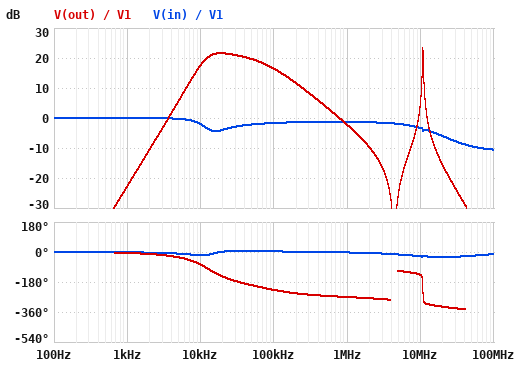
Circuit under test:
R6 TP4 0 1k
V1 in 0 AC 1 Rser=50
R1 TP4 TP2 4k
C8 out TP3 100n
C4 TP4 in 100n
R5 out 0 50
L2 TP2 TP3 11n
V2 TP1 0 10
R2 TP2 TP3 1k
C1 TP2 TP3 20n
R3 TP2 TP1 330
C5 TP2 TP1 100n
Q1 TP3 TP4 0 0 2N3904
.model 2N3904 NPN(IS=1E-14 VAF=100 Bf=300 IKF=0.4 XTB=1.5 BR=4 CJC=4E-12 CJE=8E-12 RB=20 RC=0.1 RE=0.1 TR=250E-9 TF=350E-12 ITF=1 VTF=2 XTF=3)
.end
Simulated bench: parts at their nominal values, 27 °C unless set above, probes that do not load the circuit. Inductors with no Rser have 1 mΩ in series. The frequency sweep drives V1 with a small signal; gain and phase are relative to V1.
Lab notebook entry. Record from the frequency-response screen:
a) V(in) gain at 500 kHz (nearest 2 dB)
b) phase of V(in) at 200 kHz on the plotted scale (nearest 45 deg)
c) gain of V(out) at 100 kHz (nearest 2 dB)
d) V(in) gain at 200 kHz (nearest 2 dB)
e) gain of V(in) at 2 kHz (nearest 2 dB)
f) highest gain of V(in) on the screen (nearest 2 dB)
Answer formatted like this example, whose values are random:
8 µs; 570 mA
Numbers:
-2 dB; 0 deg; 16 dB; -2 dB; 0 dB; 0 dB
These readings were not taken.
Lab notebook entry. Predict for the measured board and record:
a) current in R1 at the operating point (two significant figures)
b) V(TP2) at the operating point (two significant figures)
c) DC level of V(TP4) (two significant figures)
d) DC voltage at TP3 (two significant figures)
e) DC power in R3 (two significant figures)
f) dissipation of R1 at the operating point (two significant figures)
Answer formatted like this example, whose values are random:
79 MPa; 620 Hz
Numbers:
790 µA; 3.9 V; 730 mV; 3.9 V; 110 mW; 2.5 mW
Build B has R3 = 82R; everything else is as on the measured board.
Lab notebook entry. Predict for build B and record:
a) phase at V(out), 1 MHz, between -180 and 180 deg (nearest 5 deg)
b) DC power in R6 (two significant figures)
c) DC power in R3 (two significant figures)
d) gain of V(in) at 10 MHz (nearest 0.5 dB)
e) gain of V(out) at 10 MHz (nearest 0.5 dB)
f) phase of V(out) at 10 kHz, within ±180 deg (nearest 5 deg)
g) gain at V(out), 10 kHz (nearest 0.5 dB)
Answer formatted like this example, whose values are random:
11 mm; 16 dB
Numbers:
85 deg; 600 µW; 330 mW; -7.5 dB; 9.0 dB; -60 deg; 15.0 dB
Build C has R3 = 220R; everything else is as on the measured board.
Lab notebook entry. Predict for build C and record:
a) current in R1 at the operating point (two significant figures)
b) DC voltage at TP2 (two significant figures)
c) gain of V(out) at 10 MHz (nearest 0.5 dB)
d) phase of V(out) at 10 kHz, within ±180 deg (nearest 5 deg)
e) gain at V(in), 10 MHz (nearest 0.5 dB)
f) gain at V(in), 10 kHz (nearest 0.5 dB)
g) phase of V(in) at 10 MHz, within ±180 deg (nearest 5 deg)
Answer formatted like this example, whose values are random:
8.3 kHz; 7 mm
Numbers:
830 µA; 4.1 V; 7.5 dB; -65 deg; -4.5 dB; -1.5 dB; -30 deg
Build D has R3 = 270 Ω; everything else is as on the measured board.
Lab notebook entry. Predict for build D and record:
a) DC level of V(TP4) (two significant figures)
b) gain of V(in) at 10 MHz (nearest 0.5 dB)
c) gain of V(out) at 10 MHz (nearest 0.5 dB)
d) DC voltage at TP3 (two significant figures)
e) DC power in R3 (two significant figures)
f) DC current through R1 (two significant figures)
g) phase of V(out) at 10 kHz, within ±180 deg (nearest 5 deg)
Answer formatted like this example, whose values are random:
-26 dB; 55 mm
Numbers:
740 mV; -4.0 dB; 6.5 dB; 4.0 V; 130 mW; 810 µA; -70 deg
